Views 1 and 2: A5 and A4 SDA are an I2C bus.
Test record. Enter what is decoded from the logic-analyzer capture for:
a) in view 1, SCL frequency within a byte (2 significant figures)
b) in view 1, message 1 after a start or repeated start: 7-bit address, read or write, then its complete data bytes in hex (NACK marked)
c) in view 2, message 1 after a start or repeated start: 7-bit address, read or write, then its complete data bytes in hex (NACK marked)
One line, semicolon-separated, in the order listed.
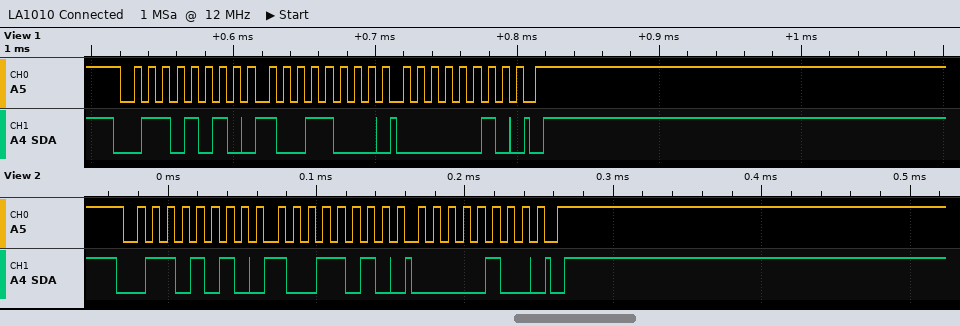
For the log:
100 kHz; 0x35 write: 98 02; 0x35 write: 9A 04
